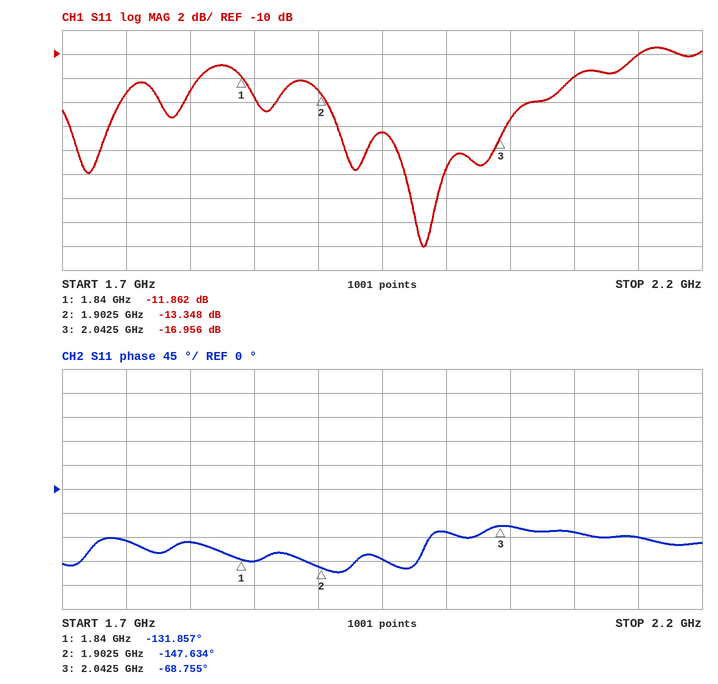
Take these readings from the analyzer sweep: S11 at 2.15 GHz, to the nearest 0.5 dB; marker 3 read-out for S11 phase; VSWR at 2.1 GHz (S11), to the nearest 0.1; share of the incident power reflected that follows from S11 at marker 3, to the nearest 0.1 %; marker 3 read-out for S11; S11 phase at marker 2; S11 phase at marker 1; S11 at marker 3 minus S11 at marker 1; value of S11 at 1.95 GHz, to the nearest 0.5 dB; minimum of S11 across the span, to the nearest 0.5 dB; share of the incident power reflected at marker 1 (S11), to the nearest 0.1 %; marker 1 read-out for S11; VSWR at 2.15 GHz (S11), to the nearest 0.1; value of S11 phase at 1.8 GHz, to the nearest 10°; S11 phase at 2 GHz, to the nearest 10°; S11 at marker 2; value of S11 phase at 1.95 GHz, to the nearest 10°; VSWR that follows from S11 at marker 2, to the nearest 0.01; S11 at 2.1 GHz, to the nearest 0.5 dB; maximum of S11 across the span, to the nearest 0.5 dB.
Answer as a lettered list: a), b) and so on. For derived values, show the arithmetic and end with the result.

a) -10.0 dB
b) -68.755°
c) |Γ| = 10^(-12/20) = 0.2512; VSWR = (1 + 0.2512)/(1 − 0.2512) ≈ 1.7
d) 10^(-16.956/10) ≈ 2.0 %
e) -16.956 dB
f) -147.634°
g) -131.857°
h) -16.956 − (-11.862) = -5.094 dB
i) -16.5 dB
j) -26.0 dB
k) 10^(-11.862/10) ≈ 6.5 %
l) -11.862 dB
m) |Γ| = 10^(-10/20) = 0.3162; VSWR = (1 + 0.3162)/(1 − 0.3162) ≈ 1.9
n) -100°
o) -80°
p) -13.348 dB
q) -130°
r) (1 + 0.2151)/(1 − 0.2151) ≈ 1.55
s) -12.0 dB
t) -9.5 dB
